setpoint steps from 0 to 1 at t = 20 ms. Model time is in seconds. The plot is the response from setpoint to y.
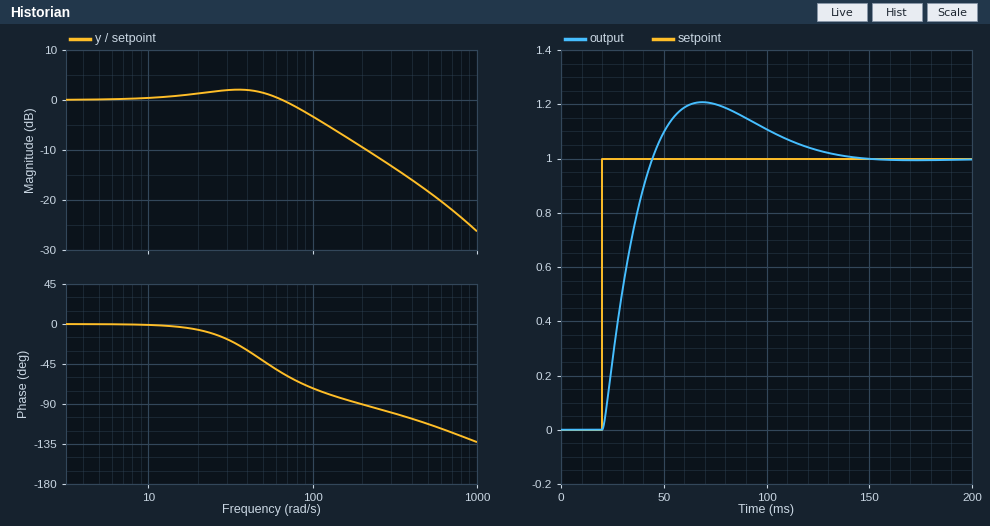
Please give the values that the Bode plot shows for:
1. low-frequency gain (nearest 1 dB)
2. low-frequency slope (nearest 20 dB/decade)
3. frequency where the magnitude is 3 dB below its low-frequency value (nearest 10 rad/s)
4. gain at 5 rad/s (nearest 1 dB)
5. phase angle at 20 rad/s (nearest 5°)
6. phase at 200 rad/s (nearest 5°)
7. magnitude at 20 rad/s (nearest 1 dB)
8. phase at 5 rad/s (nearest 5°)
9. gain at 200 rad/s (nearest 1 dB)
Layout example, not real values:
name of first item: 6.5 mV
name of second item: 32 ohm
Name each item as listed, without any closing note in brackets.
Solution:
low-frequency gain: 0 dB
low-frequency slope: 0 dB/decade
frequency where the magnitude is 3 dB below its low-frequency value: 100 rad/s
gain at 5 rad/s: 0 dB
phase angle at 20 rad/s: -5°
phase at 200 rad/s: -90°
magnitude at 20 rad/s: 1 dB
phase at 5 rad/s: 0°
gain at 200 rad/s: -9 dB
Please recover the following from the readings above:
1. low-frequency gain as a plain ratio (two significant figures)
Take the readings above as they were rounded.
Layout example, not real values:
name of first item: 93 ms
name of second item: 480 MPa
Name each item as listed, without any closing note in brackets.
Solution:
low-frequency gain as a plain ratio: 1.0
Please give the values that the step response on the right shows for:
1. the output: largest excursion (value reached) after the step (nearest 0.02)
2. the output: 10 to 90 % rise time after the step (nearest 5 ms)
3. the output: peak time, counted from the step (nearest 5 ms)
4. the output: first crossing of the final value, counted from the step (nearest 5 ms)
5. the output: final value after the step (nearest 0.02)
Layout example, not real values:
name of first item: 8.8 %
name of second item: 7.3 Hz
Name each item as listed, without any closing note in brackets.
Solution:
the output: largest excursion (value reached) after the step: 1.20
the output: 10 to 90 % rise time after the step: 20 ms
the output: peak time, counted from the step: 50 ms
the output: first crossing of the final value, counted from the step: 25 ms
the output: final value after the step: 1.00
